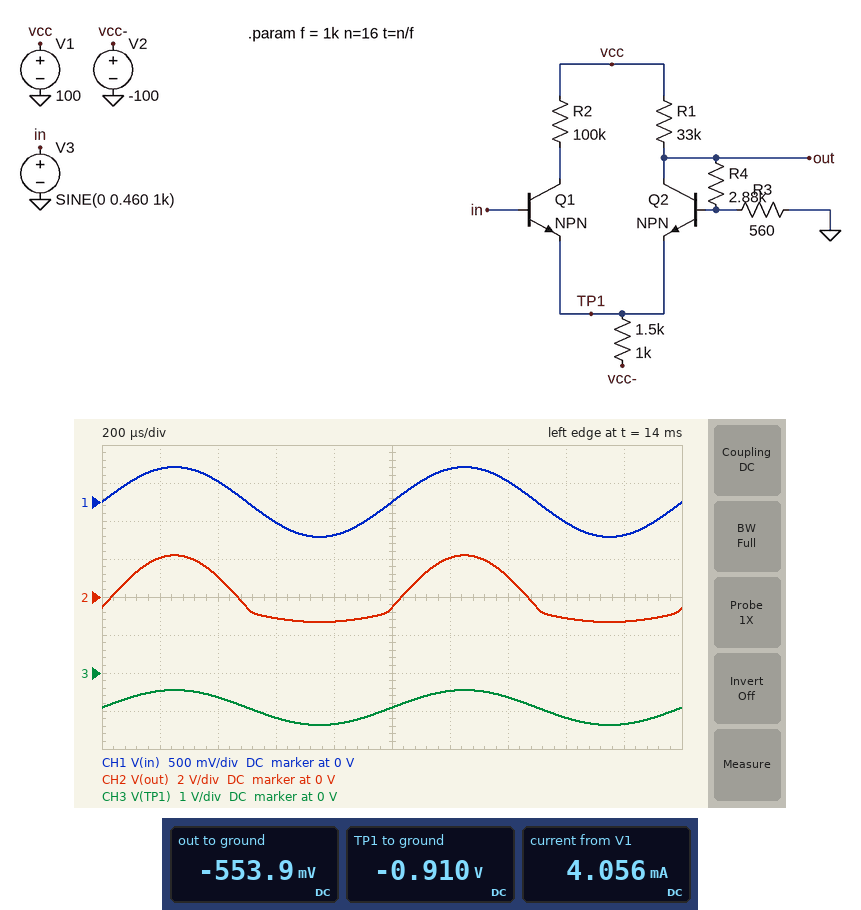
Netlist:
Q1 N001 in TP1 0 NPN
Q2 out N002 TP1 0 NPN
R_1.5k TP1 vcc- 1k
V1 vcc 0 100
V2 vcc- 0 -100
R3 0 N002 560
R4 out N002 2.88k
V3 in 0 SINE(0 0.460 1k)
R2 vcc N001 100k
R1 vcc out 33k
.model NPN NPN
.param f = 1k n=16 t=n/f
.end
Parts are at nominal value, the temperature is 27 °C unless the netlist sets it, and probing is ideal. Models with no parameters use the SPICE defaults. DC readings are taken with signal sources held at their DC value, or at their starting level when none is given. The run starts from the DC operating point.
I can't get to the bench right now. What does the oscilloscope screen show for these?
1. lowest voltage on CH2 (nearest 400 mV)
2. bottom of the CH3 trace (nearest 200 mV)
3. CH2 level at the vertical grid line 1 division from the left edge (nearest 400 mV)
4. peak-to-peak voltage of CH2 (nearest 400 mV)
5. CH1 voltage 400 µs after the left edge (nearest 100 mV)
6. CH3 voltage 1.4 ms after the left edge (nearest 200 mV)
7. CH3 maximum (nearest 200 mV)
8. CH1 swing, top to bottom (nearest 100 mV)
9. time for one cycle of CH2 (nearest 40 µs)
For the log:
-1.2 V
-1.4 V
2.0 V
3.6 V
300 mV
-600 mV
-400 mV
900 mV
1.00 ms
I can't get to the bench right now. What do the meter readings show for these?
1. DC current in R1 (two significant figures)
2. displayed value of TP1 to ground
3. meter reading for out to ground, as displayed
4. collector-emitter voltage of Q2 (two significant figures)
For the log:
3.0 mA
-0.910 V
-553.9 mV
360 mV
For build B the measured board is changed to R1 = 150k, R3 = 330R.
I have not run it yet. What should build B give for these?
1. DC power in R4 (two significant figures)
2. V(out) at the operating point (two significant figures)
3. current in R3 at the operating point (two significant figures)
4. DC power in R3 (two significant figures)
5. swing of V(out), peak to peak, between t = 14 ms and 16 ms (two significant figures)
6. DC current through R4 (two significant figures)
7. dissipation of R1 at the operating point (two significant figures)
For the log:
180 µW
-850 mV
400 µA
52 µW
3.4 V
250 µA
68 mW
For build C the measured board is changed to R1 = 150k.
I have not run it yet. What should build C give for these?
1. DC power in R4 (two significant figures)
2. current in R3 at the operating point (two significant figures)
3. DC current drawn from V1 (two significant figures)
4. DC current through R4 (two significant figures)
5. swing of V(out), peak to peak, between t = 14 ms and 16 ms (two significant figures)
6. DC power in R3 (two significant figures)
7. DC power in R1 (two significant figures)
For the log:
150 µW
250 µA
1.7 mA
230 µA
3.0 V
34 µW
68 mW
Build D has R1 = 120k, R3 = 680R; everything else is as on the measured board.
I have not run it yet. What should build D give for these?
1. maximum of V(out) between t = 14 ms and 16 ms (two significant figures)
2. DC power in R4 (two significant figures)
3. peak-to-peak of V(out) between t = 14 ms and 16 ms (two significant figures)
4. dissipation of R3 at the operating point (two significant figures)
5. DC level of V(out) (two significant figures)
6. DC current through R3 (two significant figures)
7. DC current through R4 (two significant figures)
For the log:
1.6 V
100 µW
2.9 V
27 µW
-680 mV
200 µA
190 µA
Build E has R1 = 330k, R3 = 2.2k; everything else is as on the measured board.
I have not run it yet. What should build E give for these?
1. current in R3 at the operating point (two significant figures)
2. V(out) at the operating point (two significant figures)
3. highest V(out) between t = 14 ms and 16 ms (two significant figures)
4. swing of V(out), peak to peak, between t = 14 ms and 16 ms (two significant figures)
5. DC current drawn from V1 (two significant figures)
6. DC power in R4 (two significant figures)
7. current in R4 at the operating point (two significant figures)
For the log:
73 µA
-360 mV
650 mV
1.9 V
1.3 mA
14 µW
70 µA
